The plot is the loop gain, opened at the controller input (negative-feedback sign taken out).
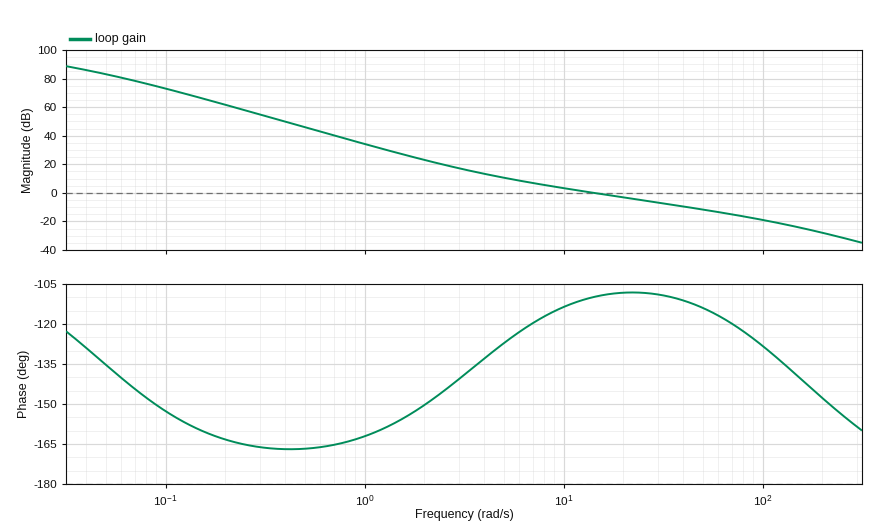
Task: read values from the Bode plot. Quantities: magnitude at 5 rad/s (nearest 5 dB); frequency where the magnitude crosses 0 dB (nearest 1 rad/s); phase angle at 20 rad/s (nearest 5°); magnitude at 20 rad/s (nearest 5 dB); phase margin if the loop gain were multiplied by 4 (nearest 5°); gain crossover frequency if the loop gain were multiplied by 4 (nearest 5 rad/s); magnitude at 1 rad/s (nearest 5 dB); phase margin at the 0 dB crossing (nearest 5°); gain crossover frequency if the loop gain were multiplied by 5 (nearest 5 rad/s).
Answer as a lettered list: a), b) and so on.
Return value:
a) 10 dB
b) 14 rad/s
c) -110°
d) -5 dB
e) 65°
f) 50 rad/s
g) 35 dB
h) 70°
i) 65 rad/s
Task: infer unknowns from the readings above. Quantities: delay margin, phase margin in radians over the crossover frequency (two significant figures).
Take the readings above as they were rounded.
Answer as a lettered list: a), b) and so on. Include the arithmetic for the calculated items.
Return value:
a) 70 × π / 180 / 14 = 0.087 s
